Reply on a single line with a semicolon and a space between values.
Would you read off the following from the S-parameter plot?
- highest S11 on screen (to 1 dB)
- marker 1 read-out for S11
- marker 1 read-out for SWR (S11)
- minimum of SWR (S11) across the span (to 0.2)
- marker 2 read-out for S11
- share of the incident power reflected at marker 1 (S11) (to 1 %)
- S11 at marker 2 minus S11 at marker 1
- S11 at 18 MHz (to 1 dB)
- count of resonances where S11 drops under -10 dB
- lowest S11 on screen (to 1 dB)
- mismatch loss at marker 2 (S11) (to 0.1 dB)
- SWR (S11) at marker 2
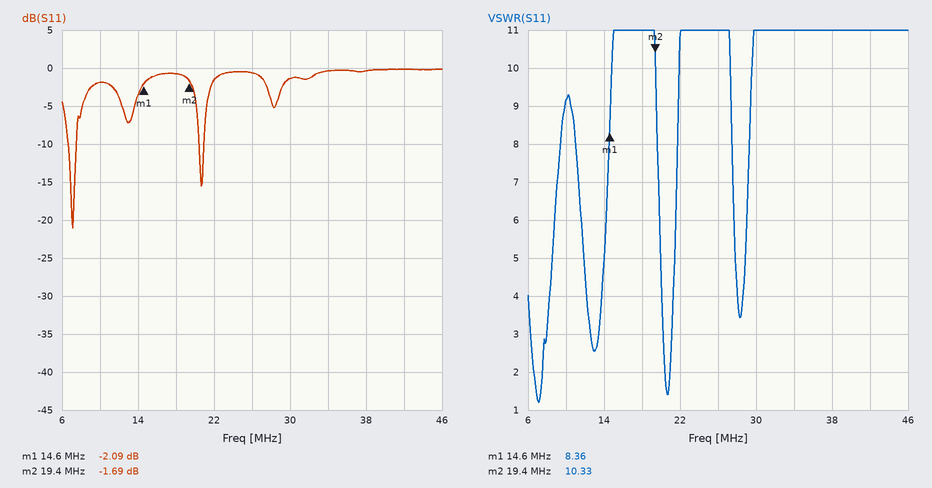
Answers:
0 dB; -2.09 dB; 8.36; 1.2; -1.69 dB; 62 %; 0.40 dB; -1 dB; 2; -21 dB; 4.9 dB; 10.33
